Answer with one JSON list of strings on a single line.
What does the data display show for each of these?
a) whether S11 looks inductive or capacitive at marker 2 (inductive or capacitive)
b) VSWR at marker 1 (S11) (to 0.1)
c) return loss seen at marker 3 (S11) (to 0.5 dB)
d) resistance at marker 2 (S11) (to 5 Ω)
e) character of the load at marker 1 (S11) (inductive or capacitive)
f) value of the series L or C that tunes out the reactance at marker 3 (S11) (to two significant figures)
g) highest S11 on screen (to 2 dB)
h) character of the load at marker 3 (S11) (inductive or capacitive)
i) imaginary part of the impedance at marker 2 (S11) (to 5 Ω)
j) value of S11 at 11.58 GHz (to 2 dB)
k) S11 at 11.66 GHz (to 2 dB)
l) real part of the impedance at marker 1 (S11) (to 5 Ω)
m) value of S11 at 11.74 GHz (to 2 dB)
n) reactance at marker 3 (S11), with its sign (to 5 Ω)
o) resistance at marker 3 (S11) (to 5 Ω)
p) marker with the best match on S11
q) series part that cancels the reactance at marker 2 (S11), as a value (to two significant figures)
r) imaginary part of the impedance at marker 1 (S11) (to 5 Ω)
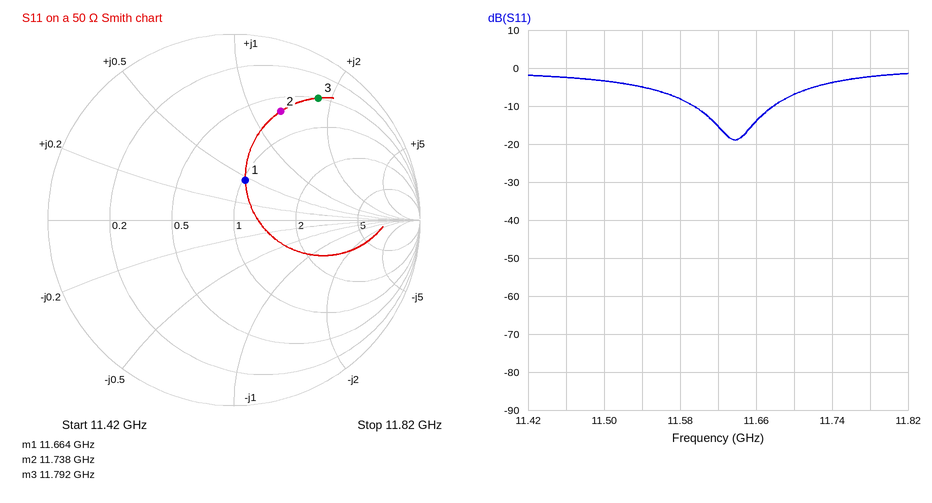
["inductive", "1.6", "2.0 dB", "35 Ω", "inductive", "150 fF", "-2 dB", "inductive", "+65 Ω", "-8 dB", "-14 dB", "50 Ω", "-4 dB", "+90 Ω", "25 Ω", "marker 1", "210 fF", "+25 Ω"]
